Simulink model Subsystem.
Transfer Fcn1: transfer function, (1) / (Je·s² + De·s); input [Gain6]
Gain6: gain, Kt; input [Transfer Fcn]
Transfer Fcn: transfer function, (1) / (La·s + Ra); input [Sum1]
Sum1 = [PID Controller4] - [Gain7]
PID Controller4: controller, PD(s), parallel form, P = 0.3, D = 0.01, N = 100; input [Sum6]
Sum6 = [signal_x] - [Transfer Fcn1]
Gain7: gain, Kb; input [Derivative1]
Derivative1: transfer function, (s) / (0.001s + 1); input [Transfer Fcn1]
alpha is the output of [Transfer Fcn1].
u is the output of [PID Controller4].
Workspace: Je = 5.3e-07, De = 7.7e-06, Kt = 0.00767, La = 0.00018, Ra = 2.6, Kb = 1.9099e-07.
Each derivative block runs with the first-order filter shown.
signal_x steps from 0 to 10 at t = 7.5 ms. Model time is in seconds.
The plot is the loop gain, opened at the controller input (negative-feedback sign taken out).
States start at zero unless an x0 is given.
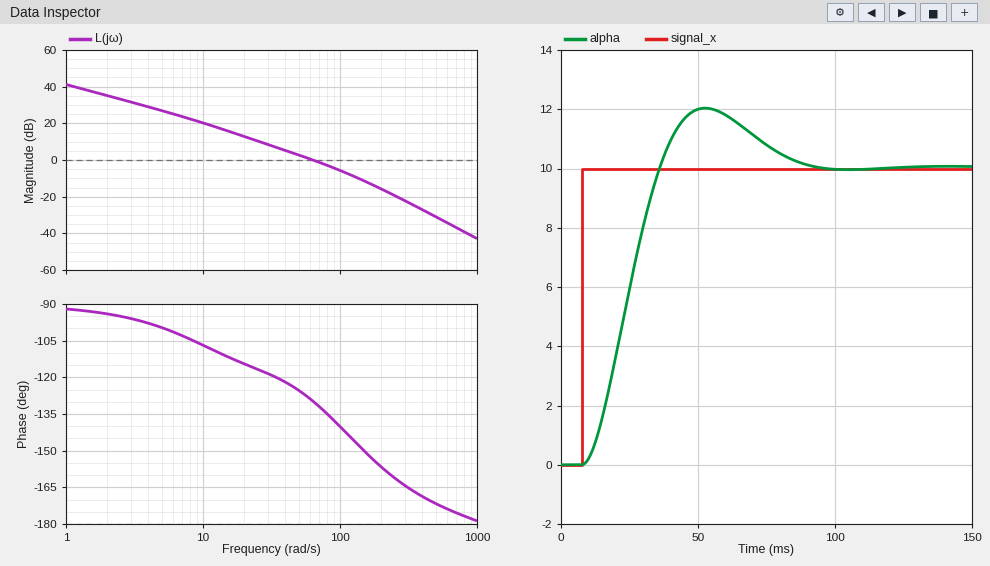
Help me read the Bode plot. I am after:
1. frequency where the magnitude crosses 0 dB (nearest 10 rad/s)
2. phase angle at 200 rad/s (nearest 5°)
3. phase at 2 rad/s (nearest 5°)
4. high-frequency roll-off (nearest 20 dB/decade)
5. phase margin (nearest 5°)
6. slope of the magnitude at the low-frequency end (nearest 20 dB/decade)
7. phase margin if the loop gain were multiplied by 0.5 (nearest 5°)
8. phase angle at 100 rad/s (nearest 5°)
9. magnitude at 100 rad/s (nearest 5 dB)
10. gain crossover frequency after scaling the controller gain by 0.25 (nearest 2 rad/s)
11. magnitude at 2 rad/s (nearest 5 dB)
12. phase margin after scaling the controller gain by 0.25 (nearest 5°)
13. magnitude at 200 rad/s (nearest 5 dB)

60 rad/s
-155°
-95°
-40 dB/decade
50°
-20 dB/decade
60°
-140°
-5 dB
22 rad/s
35 dB
65°
-15 dB
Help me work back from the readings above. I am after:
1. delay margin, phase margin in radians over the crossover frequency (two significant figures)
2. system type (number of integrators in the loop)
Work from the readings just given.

0.015 s
1
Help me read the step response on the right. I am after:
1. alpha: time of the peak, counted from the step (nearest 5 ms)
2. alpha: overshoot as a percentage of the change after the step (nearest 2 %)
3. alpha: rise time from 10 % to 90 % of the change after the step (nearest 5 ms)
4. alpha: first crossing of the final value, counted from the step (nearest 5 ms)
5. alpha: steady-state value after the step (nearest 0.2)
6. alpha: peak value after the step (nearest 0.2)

45 ms
20 %
20 ms
30 ms
10.0
12.0
